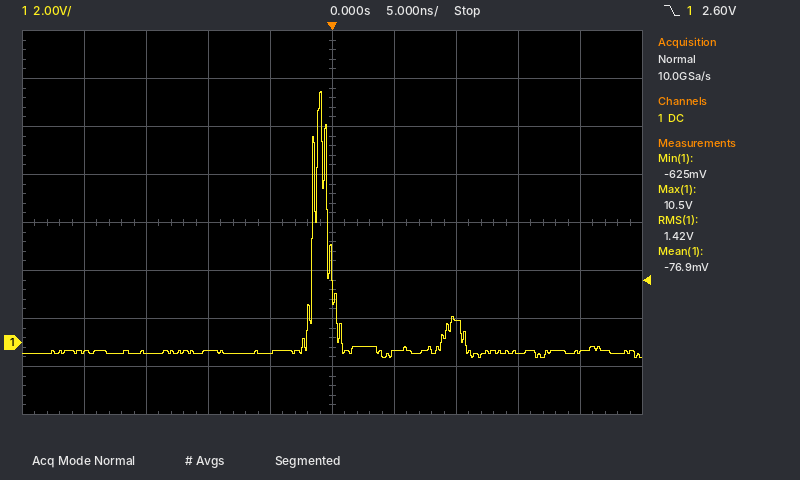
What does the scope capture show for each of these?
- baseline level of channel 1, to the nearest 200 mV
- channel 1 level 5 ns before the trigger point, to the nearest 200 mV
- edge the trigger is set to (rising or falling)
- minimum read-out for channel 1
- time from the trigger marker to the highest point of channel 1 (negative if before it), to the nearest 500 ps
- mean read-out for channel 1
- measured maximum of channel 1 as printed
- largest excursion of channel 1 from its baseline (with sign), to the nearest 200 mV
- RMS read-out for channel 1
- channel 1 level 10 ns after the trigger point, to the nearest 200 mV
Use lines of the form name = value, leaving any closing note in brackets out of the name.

baseline level of channel 1, to the nearest 200 mV = -400 mV
channel 1 level 5 ns before the trigger point, to the nearest 200 mV = -400 mV
edge the trigger is set to = falling
minimum read-out for channel 1 = -625 mV
time from the trigger marker to the highest point of channel 1 (negative if before it), to the nearest 500 ps = -1.0 ns
mean read-out for channel 1 = -76.9 mV
measured maximum of channel 1 as printed = 10.5 V
largest excursion of channel 1 from its baseline (with sign), to the nearest 200 mV = +10.8 V
RMS read-out for channel 1 = 1.42 V
channel 1 level 10 ns after the trigger point, to the nearest 200 mV = 1.0 V
